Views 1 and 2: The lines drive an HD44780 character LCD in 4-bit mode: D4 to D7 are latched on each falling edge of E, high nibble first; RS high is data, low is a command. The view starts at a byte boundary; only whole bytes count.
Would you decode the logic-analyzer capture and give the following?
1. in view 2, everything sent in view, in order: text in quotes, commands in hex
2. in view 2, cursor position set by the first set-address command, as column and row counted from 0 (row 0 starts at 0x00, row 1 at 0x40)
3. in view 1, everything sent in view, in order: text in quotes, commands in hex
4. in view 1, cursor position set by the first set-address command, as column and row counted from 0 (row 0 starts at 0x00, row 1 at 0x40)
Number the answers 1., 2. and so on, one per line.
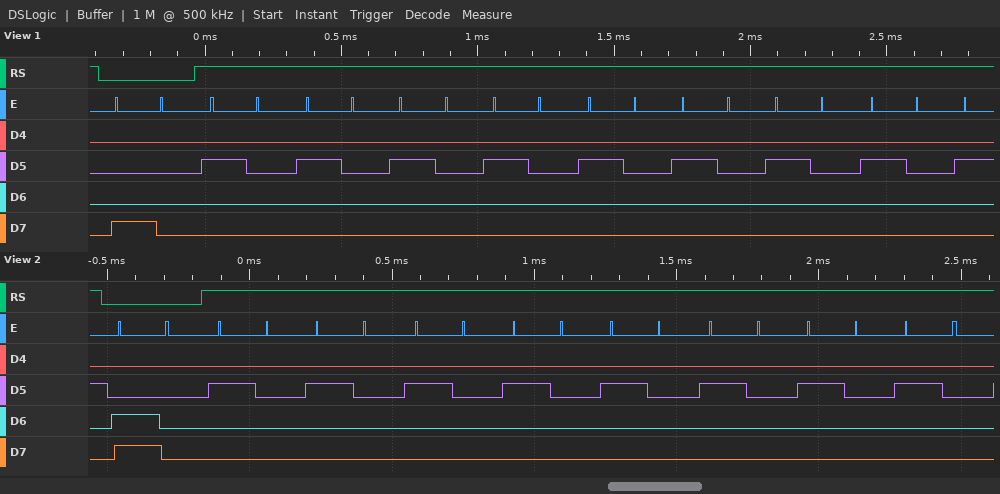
1. 0xC0 "        "
2. column 0, row 1
3. 0x80 "        "
4. column 0, row 0
